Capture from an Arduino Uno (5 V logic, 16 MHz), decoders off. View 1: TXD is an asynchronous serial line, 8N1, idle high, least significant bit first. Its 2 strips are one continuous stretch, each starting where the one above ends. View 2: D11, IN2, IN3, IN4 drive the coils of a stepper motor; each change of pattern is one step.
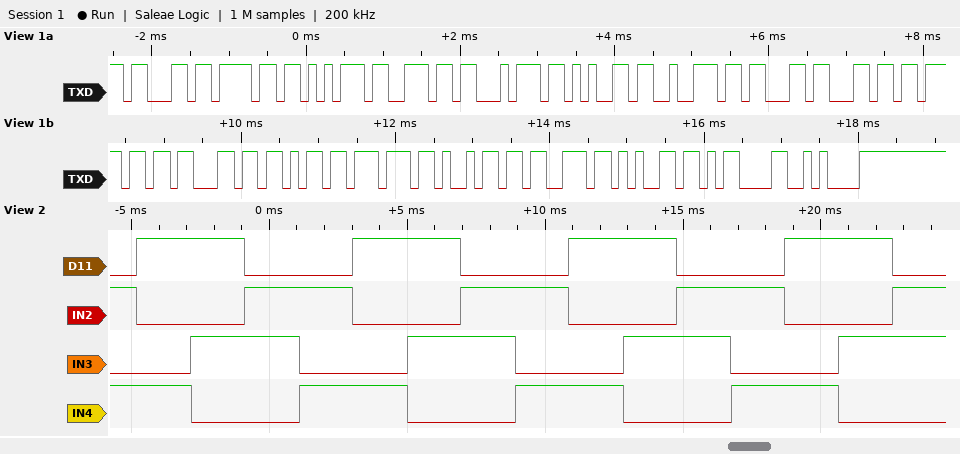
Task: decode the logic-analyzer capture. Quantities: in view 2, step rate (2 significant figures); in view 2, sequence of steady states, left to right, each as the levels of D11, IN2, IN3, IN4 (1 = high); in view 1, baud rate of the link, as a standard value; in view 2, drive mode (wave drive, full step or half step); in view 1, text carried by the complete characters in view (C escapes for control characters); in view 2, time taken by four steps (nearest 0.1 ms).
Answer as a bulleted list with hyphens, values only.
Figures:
- 510 steps/s
- 0101 1001 1010 0110 0101 1001 1010 0110 0101 1001 1010 0110 0101 1001 1010 0110
- 9600 baud
- full step
- "counterclockwise\r\n"
- 7.8 ms
